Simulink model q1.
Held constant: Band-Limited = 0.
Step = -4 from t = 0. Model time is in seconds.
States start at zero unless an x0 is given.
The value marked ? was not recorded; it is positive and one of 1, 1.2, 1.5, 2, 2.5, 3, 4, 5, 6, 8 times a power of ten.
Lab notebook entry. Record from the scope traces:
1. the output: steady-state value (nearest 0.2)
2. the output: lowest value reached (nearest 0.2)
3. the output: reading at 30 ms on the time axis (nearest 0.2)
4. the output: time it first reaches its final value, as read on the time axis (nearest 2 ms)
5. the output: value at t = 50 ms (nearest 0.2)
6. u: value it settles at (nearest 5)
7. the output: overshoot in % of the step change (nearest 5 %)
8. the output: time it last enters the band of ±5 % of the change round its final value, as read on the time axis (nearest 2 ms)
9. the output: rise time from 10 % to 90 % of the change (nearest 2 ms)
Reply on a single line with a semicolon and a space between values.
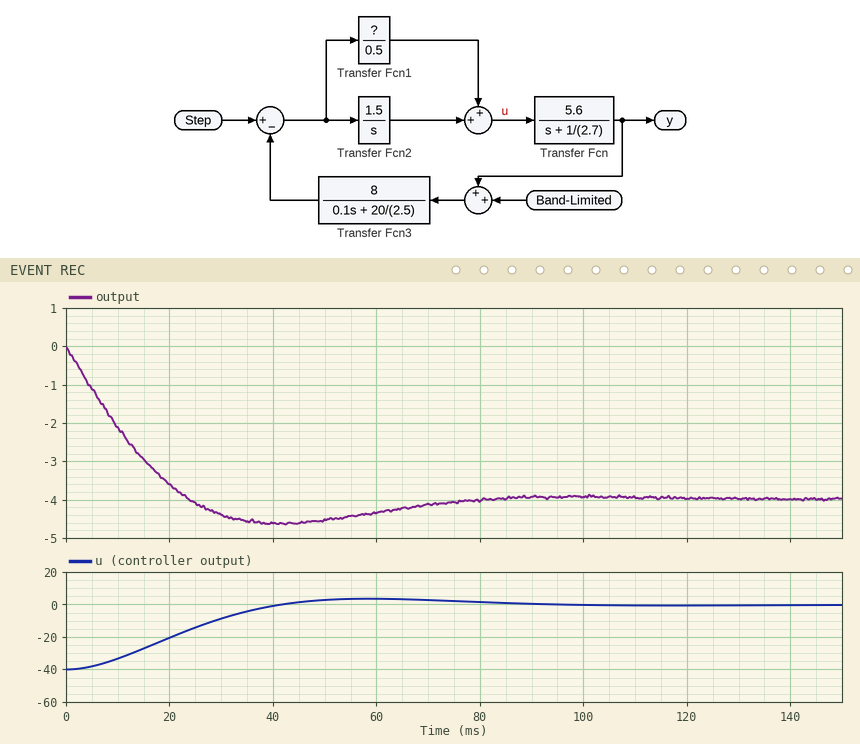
-4.0; -4.6; -4.4; 24 ms; -4.6; 0; 15 %; 68 ms; 18 ms
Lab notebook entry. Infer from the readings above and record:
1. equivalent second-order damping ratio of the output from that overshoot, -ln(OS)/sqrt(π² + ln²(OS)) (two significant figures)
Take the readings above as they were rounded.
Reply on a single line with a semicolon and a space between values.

0.52
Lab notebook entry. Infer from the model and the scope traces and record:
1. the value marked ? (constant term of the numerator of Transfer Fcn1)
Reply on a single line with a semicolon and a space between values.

5
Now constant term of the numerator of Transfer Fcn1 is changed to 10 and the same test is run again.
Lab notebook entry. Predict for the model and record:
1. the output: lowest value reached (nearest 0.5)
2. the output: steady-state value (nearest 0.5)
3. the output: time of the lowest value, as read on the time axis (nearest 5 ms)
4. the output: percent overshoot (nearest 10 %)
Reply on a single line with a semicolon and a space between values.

-6.0; -4.0; 25 ms; 50 %
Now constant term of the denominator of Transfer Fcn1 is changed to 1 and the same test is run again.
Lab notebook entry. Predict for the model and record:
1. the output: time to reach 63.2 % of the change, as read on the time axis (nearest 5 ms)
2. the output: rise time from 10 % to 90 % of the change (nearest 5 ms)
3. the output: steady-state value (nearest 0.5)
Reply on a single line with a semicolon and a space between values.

25 ms; 45 ms; -4.0
